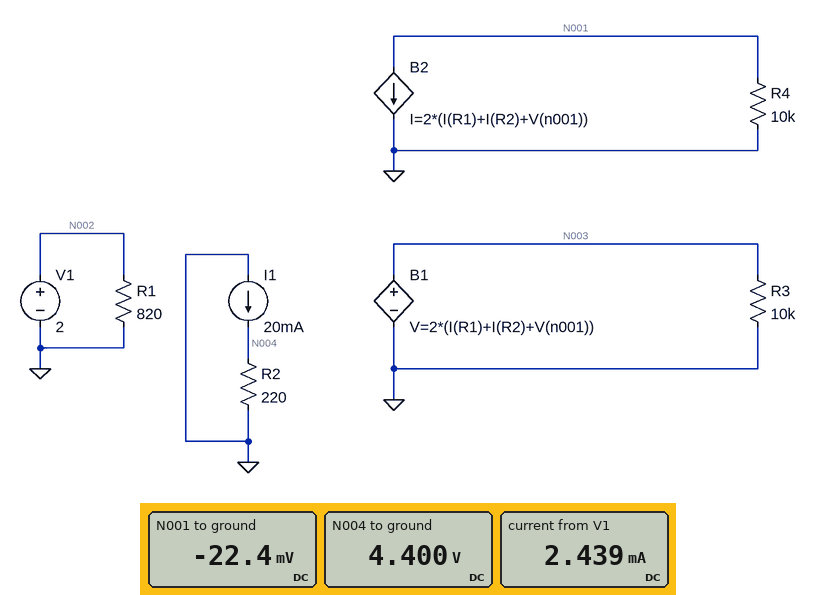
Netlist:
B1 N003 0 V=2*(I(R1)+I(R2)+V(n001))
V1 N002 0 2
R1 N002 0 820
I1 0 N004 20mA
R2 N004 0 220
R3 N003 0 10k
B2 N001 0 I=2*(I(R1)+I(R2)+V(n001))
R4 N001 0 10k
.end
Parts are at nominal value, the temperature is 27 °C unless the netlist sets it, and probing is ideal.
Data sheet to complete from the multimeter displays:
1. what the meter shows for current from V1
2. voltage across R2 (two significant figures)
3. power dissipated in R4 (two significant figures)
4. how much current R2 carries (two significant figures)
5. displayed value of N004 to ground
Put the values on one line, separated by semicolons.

2.439 mA; 4.4 V; 50 nW; 20 mA; 4.400 V
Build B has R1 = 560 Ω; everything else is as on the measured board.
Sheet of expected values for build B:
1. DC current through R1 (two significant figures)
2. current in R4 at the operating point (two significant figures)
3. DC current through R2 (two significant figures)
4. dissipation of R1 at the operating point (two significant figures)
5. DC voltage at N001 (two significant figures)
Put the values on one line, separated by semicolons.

3.6 mA; 2.4 µA; 20 mA; 7.1 mW; -24 mV
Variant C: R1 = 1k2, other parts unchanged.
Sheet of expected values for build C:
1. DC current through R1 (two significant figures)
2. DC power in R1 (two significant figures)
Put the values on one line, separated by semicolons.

1.7 mA; 3.3 mW
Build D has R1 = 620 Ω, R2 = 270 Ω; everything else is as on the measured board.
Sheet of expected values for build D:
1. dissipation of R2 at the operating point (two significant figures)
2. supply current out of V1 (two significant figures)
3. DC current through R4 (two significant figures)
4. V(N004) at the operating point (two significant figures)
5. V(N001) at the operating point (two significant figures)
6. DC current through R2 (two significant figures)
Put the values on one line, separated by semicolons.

110 mW; 3.2 mA; 2.3 µA; 5.4 V; -23 mV; 20 mA
